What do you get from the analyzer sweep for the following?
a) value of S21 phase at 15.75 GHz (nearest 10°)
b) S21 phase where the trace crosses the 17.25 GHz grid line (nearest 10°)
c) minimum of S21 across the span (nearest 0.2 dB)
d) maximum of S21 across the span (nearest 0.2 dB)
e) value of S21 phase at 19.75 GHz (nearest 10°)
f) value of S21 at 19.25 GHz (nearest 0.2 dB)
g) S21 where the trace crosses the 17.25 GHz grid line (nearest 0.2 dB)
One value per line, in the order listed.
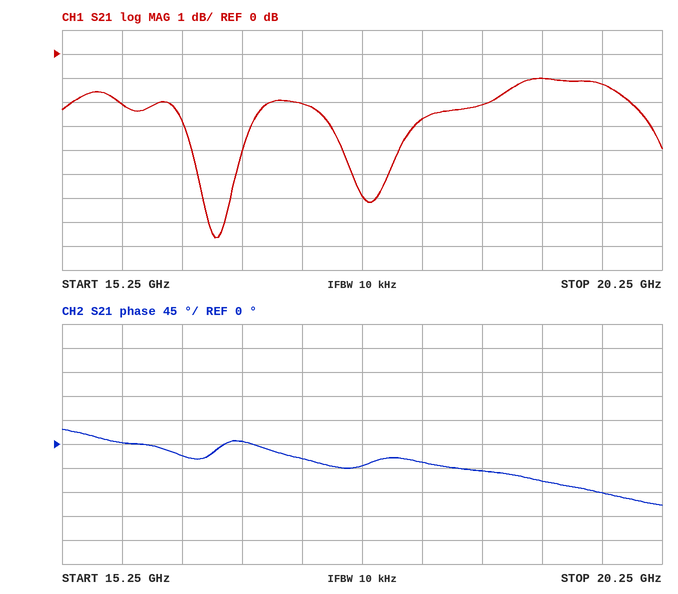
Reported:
0°
-30°
-7.6 dB
-1.0 dB
-90°
-1.0 dB
-2.0 dB
